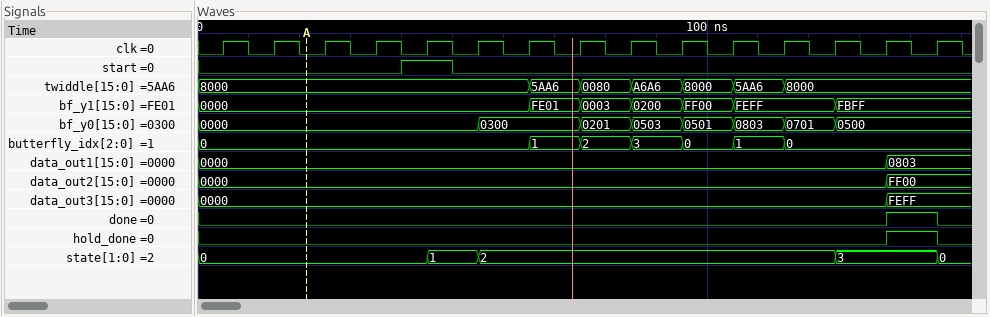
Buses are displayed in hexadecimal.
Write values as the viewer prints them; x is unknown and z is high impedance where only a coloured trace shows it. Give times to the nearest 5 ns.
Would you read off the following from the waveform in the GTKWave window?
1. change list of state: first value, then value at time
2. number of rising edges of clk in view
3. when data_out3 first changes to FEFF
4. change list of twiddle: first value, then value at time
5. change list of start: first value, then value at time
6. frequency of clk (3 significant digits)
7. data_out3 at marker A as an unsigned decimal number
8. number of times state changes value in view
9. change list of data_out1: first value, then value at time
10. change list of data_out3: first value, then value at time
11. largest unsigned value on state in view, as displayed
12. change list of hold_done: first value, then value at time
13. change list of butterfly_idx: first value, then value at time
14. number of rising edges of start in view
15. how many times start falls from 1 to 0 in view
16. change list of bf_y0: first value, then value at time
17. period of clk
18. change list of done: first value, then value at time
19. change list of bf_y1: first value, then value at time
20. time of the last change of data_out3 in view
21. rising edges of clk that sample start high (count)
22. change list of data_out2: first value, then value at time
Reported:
0, 1 at 45 ns, 2 at 55 ns, 3 at 125 ns, 0 at 145 ns
15
135 ns
8000, 5AA6 at 65 ns, 0080 at 75 ns, A6A6 at 85 ns, 8000 at 95 ns, 5AA6 at 105 ns, 8000 at 115 ns
0, 1 at 40 ns, 0 at 50 ns
100 MHz
0
4
0000, 0803 at 135 ns
0000, FEFF at 135 ns
3
0, 1 at 135 ns, 0 at 145 ns
0, 1 at 65 ns, 2 at 75 ns, 3 at 85 ns, 0 at 95 ns, 1 at 105 ns, 0 at 115 ns
1
1
0000, 0300 at 55 ns, 0201 at 75 ns, 0503 at 85 ns, 0501 at 95 ns, 0803 at 105 ns, 0701 at 115 ns, 0500 at 125 ns
10 ns
0, 1 at 135 ns, 0 at 145 ns
0000, FE01 at 65 ns, 0003 at 75 ns, 0200 at 85 ns, FF00 at 95 ns, FEFF at 105 ns, FBFF at 125 ns
135 ns
1
0000, FF00 at 135 ns
